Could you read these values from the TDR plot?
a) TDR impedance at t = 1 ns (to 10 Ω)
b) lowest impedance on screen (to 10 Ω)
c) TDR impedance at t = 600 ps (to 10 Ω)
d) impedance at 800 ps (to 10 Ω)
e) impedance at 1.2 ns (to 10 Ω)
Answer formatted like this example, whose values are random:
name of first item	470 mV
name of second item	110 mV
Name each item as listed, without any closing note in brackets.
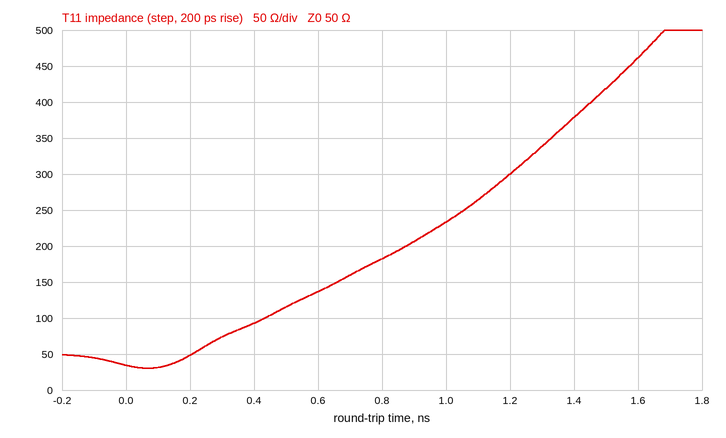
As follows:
TDR impedance at t = 1 ns	230 Ω
lowest impedance on screen	30 Ω
TDR impedance at t = 600 ps	140 Ω
impedance at 800 ps	180 Ω
impedance at 1.2 ns	300 Ω
